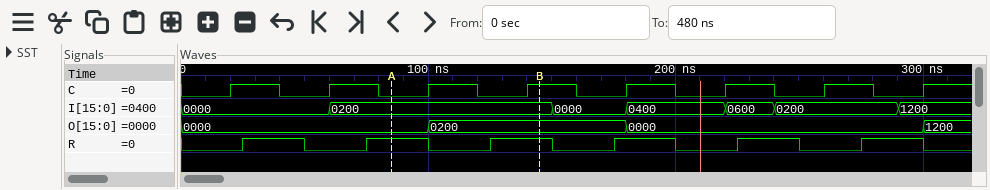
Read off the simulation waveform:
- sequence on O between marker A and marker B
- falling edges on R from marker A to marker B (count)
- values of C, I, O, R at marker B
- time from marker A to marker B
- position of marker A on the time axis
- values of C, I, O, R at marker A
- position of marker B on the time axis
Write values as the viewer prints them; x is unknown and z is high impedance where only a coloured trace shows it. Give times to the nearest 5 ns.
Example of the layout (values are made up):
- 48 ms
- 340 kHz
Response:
- 0000, 0200
- 1
- C=1, I=0200, O=0200, R=1
- 60 ns
- 85 ns
- C=0, I=0200, O=0000, R=1
- 145 ns
